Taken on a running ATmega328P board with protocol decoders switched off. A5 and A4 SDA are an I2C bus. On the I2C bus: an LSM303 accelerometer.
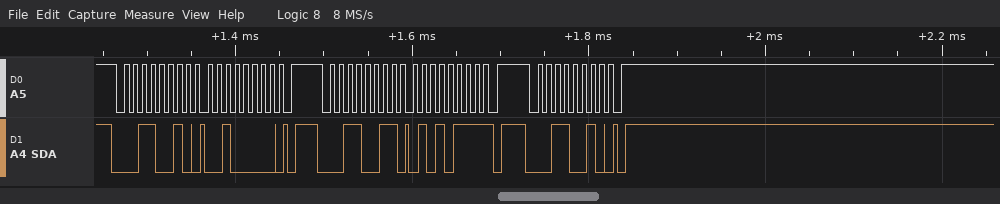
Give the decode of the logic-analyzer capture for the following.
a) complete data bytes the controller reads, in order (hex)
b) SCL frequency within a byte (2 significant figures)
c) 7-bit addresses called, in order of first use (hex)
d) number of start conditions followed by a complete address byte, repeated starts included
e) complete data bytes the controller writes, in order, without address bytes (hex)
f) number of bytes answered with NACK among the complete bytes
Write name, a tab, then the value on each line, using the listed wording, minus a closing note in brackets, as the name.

complete data bytes the controller reads, in order	57
SCL frequency within a byte	100 kHz
7-bit addresses called, in order of first use	0x19
number of start conditions followed by a complete address byte, repeated starts included	3
complete data bytes the controller writes, in order, without address bytes	20
number of bytes answered with NACK among the complete bytes	1
